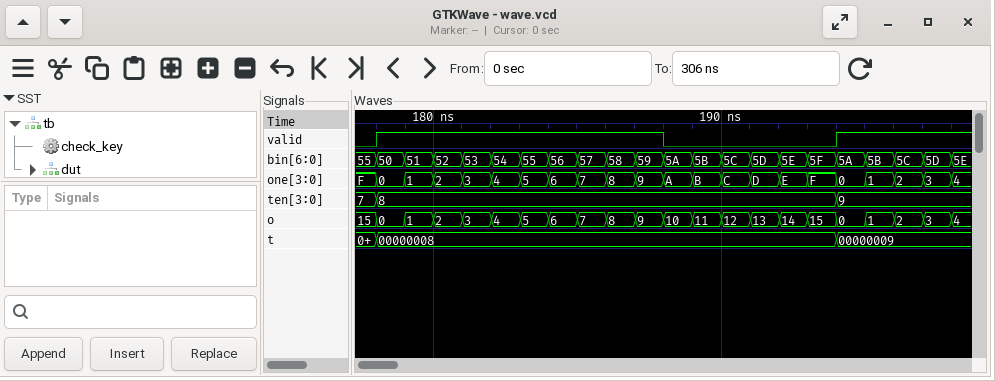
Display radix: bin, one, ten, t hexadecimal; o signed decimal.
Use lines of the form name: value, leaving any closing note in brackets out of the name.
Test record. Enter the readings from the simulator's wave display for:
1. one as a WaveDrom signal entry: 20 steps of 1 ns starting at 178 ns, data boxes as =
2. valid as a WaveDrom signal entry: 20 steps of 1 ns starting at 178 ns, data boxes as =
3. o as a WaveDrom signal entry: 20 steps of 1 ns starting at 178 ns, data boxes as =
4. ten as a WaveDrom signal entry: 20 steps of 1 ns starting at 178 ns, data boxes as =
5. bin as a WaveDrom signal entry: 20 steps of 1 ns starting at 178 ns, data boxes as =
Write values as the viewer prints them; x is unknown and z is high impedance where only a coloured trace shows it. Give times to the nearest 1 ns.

one as a WaveDrom signal entry: 20 steps of 1 ns starting at 178 ns, data boxes as =: {name: 'one', wave: '====================', data: '0 1 2 3 4 5 6 7 8 9 A B C D E F 0 1 2 3'}
valid as a WaveDrom signal entry: 20 steps of 1 ns starting at 178 ns, data boxes as =: {name: 'valid', wave: '1.........0.....1...'}
o as a WaveDrom signal entry: 20 steps of 1 ns starting at 178 ns, data boxes as =: {name: 'o', wave: '====================', data: '0 1 2 3 4 5 6 7 8 9 10 11 12 13 14 15 0 1 2 3'}
ten as a WaveDrom signal entry: 20 steps of 1 ns starting at 178 ns, data boxes as =: {name: 'ten', wave: '=...............=...', data: '8 9'}
bin as a WaveDrom signal entry: 20 steps of 1 ns starting at 178 ns, data boxes as =: {name: 'bin', wave: '====================', data: '50 51 52 53 54 55 56 57 58 59 5A 5B 5C 5D 5E 5F 5A 5B 5C 5D'}
